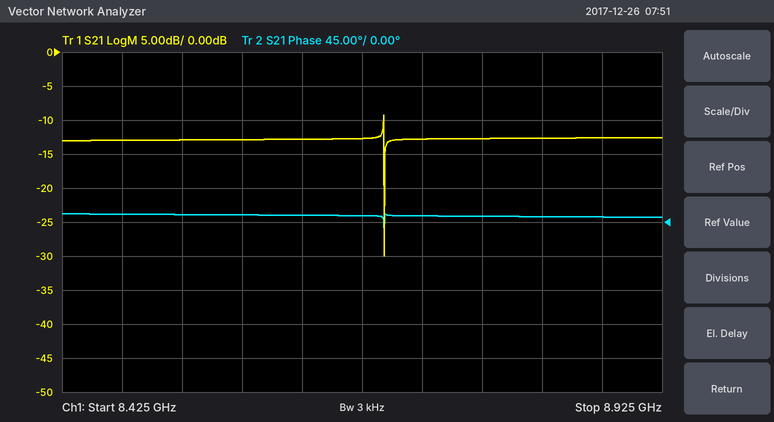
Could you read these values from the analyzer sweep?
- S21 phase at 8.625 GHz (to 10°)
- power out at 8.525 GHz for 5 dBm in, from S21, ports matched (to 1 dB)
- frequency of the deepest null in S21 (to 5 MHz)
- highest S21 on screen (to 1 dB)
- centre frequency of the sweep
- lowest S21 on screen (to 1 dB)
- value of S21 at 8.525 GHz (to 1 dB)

10°
-8 dBm
8.695 GHz
-9 dB
8.675 GHz
-30 dB
-13 dB
